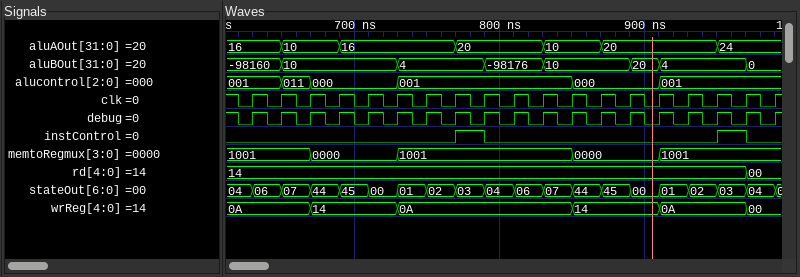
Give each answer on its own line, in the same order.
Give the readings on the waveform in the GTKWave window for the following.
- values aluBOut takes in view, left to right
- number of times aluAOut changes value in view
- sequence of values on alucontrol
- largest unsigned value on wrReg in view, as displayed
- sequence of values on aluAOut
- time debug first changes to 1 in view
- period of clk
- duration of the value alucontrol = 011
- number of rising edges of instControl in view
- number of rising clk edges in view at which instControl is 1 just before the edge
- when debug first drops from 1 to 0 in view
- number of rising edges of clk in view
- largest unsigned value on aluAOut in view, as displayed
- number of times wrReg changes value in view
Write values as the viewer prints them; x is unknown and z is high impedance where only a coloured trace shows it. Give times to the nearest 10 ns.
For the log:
-98160, 10, 4, -98176, 10, 20, 4, 0
6
001, 011, 000, 001, 000, 001
14
16, 10, 16, 20, 10, 20, 24
630 ns
20 ns
20 ns
2
2
620 ns
19
24
5
